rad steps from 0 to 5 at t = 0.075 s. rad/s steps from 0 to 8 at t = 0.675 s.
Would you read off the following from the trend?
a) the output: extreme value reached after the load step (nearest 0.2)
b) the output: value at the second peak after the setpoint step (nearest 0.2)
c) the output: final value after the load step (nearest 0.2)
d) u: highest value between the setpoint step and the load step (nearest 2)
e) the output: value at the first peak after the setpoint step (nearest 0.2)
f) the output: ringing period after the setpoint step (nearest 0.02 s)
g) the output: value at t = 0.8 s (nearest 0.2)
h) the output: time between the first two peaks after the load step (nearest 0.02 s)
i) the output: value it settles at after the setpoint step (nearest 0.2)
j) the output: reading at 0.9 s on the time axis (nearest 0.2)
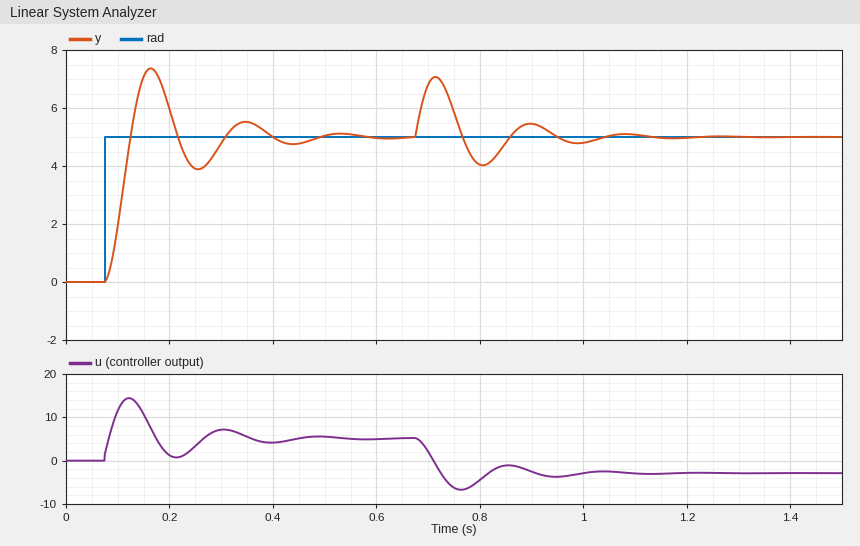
7.0
5.6
5.0
14
7.4
0.18 s
4.0
0.18 s
5.0
5.4
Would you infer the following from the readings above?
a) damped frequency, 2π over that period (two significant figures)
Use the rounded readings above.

35 rad/s
